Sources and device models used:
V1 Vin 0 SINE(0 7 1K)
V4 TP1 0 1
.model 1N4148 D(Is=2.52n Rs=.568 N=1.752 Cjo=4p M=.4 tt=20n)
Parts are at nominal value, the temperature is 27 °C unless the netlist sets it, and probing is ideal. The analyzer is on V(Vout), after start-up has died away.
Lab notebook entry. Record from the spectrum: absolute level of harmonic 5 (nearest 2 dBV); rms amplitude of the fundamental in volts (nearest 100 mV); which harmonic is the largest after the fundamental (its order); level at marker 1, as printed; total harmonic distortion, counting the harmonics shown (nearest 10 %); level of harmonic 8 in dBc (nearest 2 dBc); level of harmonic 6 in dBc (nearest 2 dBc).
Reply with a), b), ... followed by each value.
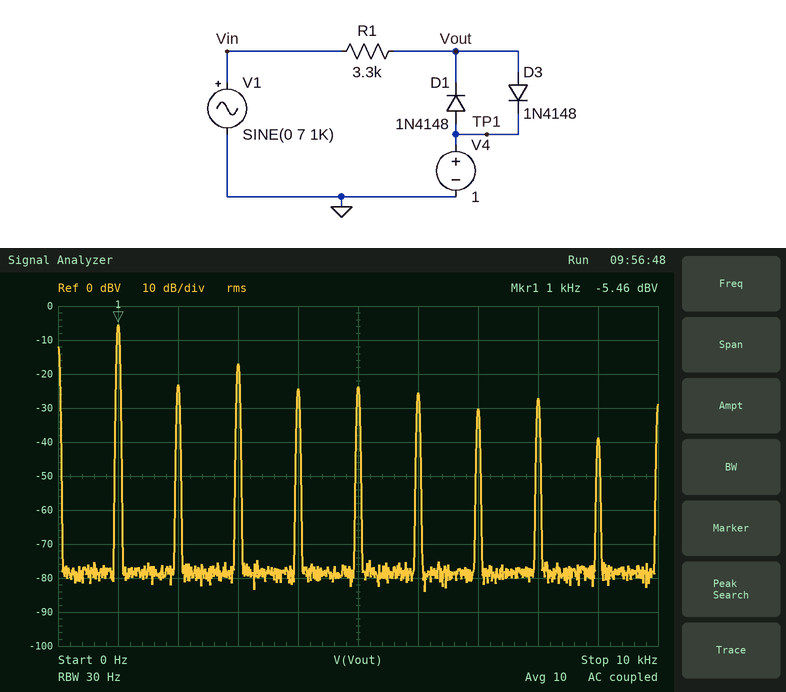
a) -24 dBV
b) 500 mV
c) 3
d) -5.46 dBV
e) 40 %
f) -22 dBc
g) -20 dBc
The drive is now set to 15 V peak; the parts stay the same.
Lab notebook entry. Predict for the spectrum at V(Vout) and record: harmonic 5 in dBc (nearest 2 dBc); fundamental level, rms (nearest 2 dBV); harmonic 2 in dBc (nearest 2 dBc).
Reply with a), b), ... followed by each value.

a) -16 dBc
b) -4 dBV
c) -24 dBc
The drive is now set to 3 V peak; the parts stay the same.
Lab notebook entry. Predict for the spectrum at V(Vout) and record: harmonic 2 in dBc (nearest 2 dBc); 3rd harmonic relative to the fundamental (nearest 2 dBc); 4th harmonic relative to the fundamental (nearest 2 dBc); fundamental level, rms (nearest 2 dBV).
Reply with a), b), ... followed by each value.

a) -10 dBc
b) -16 dBc
c) -14 dBc
d) -6 dBV
